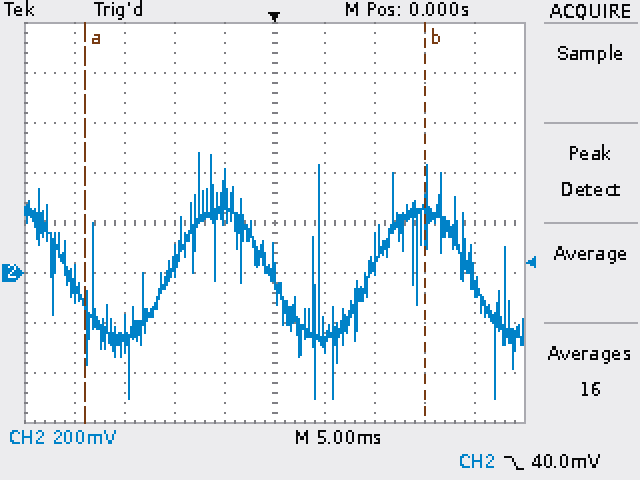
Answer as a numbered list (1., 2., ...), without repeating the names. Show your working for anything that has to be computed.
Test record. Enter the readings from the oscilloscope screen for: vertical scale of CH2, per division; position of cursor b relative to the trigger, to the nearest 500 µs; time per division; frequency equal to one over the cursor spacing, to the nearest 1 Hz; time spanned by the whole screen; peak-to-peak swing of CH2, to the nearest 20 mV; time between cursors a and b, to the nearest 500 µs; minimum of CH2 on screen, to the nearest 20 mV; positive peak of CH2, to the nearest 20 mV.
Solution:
1. 200 mV
2. +15.0 ms
3. 5 ms
4. 1 / 34.0 ms ≈ 29 Hz
5. 50 ms
6. 480 mV − (-500 mV) = 980 mV
7. 34.0 ms
8. -500 mV
9. 480 mV
